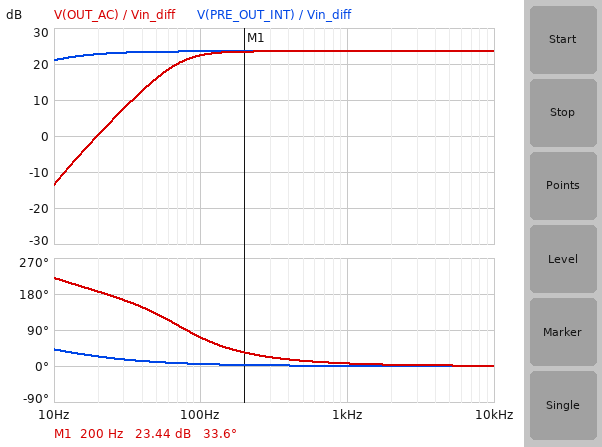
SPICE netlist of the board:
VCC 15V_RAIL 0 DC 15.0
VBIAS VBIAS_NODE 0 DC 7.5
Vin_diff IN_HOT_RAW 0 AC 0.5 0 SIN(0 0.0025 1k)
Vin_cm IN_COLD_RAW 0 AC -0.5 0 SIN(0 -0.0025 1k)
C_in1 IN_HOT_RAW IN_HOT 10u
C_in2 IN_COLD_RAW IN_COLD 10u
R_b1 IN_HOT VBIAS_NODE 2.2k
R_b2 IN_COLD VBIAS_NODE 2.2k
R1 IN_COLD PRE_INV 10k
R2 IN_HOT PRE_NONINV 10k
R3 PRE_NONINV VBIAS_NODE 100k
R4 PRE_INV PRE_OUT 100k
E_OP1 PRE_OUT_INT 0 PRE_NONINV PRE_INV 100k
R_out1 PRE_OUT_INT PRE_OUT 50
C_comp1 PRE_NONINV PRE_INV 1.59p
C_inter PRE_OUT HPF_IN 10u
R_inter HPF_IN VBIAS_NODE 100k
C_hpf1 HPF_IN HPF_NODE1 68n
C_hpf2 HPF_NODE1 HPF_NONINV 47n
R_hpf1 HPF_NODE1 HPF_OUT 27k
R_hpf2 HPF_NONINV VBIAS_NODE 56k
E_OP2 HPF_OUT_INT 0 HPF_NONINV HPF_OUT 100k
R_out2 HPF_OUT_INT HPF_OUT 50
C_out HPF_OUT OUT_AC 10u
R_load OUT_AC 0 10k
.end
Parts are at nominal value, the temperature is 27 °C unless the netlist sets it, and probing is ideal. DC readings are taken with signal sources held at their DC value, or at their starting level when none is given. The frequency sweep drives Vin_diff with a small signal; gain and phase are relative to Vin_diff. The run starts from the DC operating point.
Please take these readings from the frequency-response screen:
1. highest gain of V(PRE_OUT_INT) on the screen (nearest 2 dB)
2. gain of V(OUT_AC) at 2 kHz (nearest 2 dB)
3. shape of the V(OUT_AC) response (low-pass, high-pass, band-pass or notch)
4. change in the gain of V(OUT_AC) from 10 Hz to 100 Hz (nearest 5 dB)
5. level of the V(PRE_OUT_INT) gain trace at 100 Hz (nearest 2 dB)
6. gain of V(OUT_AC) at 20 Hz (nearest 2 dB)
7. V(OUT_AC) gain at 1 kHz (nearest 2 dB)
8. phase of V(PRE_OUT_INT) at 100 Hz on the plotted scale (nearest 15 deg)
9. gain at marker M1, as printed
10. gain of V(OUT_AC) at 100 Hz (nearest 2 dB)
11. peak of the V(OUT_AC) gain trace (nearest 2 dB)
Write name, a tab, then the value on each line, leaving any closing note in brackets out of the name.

highest gain of V(PRE_OUT_INT) on the screen	24 dB
gain of V(OUT_AC) at 2 kHz	24 dB
shape of the V(OUT_AC) response	high-pass
change in the gain of V(OUT_AC) from 10 Hz to 100 Hz	35 dB
level of the V(PRE_OUT_INT) gain trace at 100 Hz	24 dB
gain of V(OUT_AC) at 20 Hz	0 dB
V(OUT_AC) gain at 1 kHz	24 dB
phase of V(PRE_OUT_INT) at 100 Hz on the plotted scale	0 deg
gain at marker M1, as printed	23.44 dB
gain of V(OUT_AC) at 100 Hz	22 dB
peak of the V(OUT_AC) gain trace	24 dB
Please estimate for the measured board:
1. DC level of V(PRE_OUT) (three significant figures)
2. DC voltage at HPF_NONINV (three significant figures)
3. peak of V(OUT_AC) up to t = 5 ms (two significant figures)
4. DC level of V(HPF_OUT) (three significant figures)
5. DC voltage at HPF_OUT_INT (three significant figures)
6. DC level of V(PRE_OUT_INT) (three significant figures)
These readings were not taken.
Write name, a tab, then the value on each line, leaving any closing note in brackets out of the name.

DC level of V(PRE_OUT)	7.50 V
DC voltage at HPF_NONINV	7.50 V
peak of V(OUT_AC) up to t = 5 ms	50 mV
DC level of V(HPF_OUT)	7.50 V
DC voltage at HPF_OUT_INT	7.50 V
DC level of V(PRE_OUT_INT)	7.50 V
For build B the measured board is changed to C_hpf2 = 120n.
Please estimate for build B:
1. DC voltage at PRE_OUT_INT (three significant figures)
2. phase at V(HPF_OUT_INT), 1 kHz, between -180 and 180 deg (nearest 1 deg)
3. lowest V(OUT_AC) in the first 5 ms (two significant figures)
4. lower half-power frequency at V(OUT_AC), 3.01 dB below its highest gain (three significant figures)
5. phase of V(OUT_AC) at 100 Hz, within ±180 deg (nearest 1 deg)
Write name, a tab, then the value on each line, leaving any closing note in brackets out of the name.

DC voltage at PRE_OUT_INT	7.50 V
phase at V(HPF_OUT_INT), 1 kHz, between -180 and 180 deg	4 deg
lowest V(OUT_AC) in the first 5 ms	-53 mV
lower half-power frequency at V(OUT_AC), 3.01 dB below its highest gain	47.4 Hz
phase of V(OUT_AC) at 100 Hz, within ±180 deg	46 deg
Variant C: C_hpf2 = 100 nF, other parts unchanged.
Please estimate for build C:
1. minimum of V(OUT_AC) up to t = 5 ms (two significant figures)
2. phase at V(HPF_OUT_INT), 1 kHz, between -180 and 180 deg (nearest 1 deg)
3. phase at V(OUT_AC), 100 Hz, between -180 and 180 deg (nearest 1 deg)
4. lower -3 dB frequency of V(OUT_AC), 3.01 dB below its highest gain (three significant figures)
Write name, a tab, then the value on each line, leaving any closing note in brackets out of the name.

minimum of V(OUT_AC) up to t = 5 ms	-53 mV
phase at V(HPF_OUT_INT), 1 kHz, between -180 and 180 deg	5 deg
phase at V(OUT_AC), 100 Hz, between -180 and 180 deg	49 deg
lower -3 dB frequency of V(OUT_AC), 3.01 dB below its highest gain	50.6 Hz
